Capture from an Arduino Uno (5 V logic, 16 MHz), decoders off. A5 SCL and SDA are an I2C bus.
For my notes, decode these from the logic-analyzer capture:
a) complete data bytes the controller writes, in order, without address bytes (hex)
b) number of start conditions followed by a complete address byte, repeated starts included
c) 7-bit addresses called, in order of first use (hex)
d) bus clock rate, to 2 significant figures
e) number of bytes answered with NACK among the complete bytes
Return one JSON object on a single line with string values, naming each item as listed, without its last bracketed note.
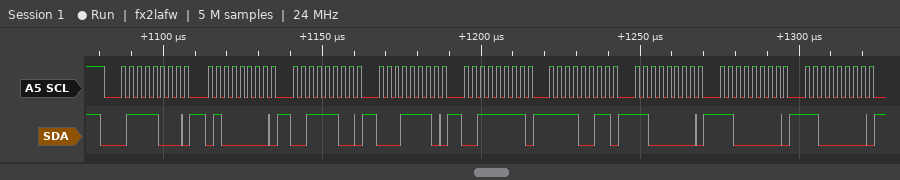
{"complete data bytes the controller writes, in order, without address bytes": "40 3C 1E 3F F3 C0 C0 C0", "number of start conditions followed by a complete address byte, repeated starts included": "1", "7-bit addresses called, in order of first use": "0x3C", "bus clock rate, to 2 significant figures": "400 kHz", "number of bytes answered with NACK among the complete bytes": "0"}
